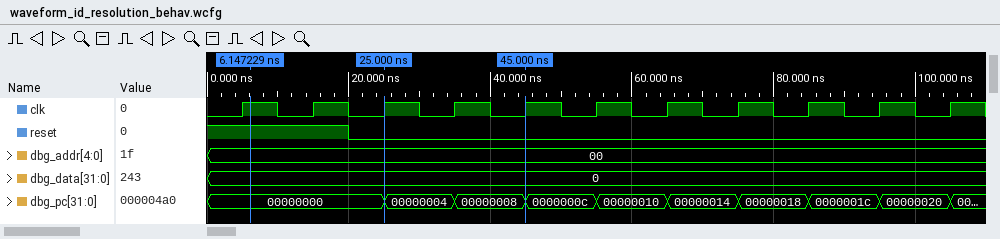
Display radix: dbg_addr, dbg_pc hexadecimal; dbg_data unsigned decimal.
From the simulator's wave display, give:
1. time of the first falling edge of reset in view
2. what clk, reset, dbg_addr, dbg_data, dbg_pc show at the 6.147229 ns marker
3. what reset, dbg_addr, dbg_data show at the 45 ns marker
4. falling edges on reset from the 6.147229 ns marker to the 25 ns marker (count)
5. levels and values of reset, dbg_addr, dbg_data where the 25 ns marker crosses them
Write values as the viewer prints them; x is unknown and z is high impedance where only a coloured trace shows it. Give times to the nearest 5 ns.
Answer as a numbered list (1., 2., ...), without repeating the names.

1. 20 ns
2. clk=1, reset=1, dbg_addr=00, dbg_data=0, dbg_pc=00000000
3. reset=0, dbg_addr=00, dbg_data=0
4. 1
5. reset=0, dbg_addr=00, dbg_data=0
